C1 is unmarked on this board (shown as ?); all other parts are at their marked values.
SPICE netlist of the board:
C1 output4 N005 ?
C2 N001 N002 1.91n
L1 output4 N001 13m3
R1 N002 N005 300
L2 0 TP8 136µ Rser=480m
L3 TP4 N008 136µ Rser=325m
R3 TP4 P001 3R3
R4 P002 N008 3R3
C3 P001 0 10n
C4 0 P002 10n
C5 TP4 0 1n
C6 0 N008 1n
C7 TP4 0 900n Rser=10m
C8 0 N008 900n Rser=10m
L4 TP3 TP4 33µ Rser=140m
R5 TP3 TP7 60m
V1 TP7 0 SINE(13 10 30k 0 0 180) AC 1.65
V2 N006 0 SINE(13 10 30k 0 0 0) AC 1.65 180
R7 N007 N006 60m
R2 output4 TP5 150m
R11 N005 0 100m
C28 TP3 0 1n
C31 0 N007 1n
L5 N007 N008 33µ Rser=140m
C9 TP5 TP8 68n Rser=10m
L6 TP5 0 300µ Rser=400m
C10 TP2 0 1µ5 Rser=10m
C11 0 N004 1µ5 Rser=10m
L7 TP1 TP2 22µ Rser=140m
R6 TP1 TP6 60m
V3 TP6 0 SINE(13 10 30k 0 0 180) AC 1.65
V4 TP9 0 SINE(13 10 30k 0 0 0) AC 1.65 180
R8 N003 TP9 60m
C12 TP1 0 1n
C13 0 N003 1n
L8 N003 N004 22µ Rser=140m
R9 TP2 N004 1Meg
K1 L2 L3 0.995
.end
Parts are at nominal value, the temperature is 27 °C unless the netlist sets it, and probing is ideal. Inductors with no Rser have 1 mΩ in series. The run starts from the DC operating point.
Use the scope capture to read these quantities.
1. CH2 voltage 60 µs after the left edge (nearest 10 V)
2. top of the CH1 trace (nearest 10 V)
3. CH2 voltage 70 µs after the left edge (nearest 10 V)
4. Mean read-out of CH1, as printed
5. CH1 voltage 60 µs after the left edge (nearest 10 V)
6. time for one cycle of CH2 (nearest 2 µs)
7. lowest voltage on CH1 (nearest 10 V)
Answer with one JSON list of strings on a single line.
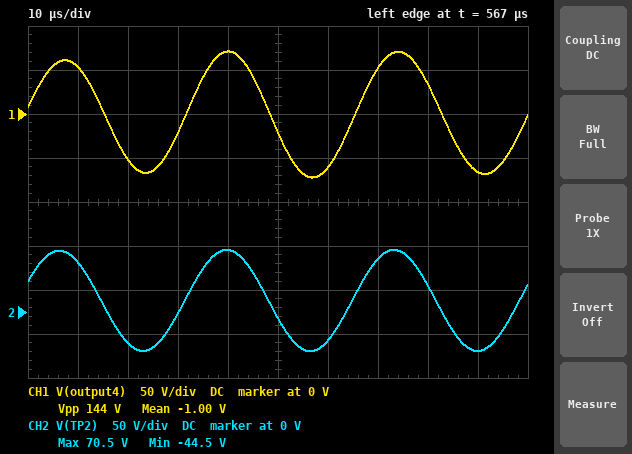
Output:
["-30 V", "70 V", "60 V", "-1.00 V", "-60 V", "34 µs", "-70 V"]
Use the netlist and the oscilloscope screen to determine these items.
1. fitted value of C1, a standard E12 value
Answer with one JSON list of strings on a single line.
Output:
["56 nF"]
